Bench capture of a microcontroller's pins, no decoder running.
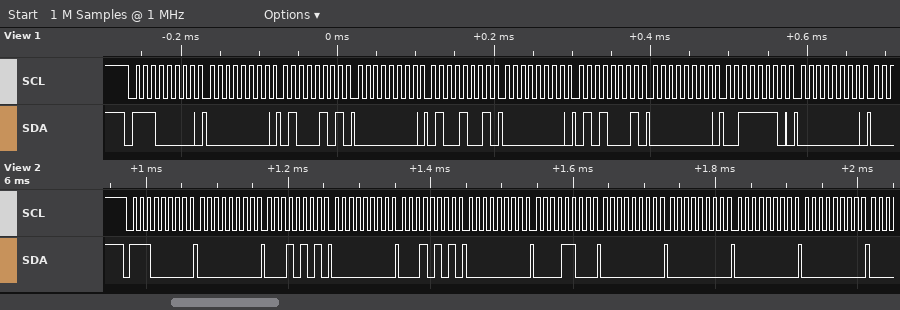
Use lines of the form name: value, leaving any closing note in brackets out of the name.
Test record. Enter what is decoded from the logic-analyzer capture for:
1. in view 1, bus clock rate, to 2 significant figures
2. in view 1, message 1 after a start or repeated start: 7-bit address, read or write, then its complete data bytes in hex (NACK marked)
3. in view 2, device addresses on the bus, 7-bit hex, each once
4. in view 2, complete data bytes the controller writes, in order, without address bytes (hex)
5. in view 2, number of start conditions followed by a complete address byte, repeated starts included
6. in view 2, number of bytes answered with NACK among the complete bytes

in view 1, bus clock rate, to 2 significant figures: 100 kHz
in view 1, message 1 after a start or repeated start: 7-bit address, read or write, then its complete data bytes in hex: 0x70 write: 00 45 00 49 00 51 00 3E 00
in view 2, device addresses on the bus, 7-bit hex, each once: 0x70
in view 2, complete data bytes the controller writes, in order, without address bytes: 00 15 00 15 00 0C 00 00 00 00
in view 2, number of start conditions followed by a complete address byte, repeated starts included: 1
in view 2, number of bytes answered with NACK among the complete bytes: 0
